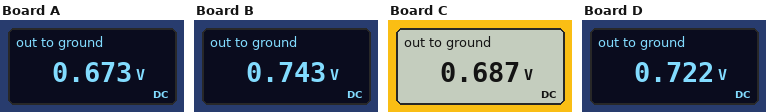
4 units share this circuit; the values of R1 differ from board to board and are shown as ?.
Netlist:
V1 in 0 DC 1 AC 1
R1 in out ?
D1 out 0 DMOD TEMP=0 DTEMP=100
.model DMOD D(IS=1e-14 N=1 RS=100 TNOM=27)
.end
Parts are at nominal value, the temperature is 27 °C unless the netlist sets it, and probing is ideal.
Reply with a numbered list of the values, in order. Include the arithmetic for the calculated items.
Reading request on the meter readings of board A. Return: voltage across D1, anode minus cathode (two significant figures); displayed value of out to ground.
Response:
1. 673 mV = 670 mV
2. 0.673 V
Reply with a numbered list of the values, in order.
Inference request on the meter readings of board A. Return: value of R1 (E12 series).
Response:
1. 2.2 kΩ
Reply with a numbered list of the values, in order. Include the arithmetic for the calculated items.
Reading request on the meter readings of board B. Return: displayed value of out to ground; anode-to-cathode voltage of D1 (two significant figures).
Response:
1. 0.743 V
2. 743 mV = 740 mV
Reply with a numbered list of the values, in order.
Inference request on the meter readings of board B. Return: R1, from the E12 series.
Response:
1. 470 Ω
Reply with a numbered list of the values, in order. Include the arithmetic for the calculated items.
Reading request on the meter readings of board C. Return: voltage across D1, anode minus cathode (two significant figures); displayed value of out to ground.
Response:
1. 687 mV = 690 mV
2. 0.687 V
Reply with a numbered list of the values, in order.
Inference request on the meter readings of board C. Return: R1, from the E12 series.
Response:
1. 1.5 kΩ
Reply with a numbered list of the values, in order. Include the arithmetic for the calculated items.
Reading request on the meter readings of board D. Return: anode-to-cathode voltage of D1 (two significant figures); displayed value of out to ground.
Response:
1. 722 mV = 720 mV
2. 0.722 V
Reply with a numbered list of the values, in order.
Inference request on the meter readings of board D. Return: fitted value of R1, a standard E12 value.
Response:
1. 680 Ω
